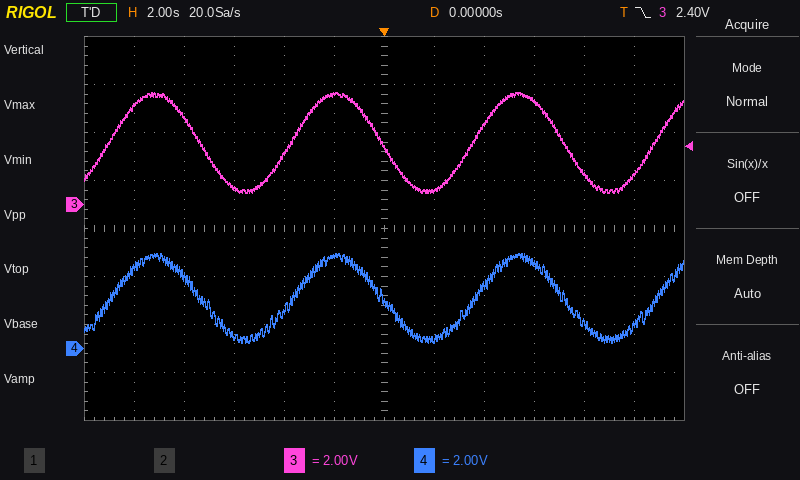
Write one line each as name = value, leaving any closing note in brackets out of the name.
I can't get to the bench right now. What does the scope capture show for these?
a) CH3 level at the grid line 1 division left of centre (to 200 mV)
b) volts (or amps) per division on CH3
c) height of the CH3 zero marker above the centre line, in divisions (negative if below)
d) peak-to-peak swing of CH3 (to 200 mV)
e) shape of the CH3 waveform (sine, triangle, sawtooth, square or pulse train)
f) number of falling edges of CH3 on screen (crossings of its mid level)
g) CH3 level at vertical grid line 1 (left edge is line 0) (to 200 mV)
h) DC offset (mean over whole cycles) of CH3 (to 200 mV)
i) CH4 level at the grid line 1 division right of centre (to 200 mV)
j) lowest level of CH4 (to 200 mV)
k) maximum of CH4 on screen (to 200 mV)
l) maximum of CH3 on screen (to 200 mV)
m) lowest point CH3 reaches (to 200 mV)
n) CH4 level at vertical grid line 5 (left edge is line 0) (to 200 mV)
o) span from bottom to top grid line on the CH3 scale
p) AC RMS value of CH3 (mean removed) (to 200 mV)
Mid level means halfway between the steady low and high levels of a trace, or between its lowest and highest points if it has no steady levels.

CH3 level at the grid line 1 division left of centre = 4.6 V
volts (or amps) per division on CH3 = 2 V
height of the CH3 zero marker above the centre line, in divisions = +0.5 div
peak-to-peak swing of CH3 = 4.2 V
shape of the CH3 waveform = sine
number of falling edges of CH3 on screen = 3
CH3 level at vertical grid line 1 (left edge is line 0) = 4.0 V
DC offset (mean over whole cycles) of CH3 = 2.6 V
CH4 level at the grid line 1 division right of centre = 400 mV
lowest level of CH4 = 200 mV
maximum of CH4 on screen = 4.0 V
maximum of CH3 on screen = 4.6 V
lowest point CH3 reaches = 400 mV
CH4 level at vertical grid line 5 (left edge is line 0) = 3.8 V
span from bottom to top grid line on the CH3 scale = 16 V
AC RMS value of CH3 (mean removed) = 1.4 V
